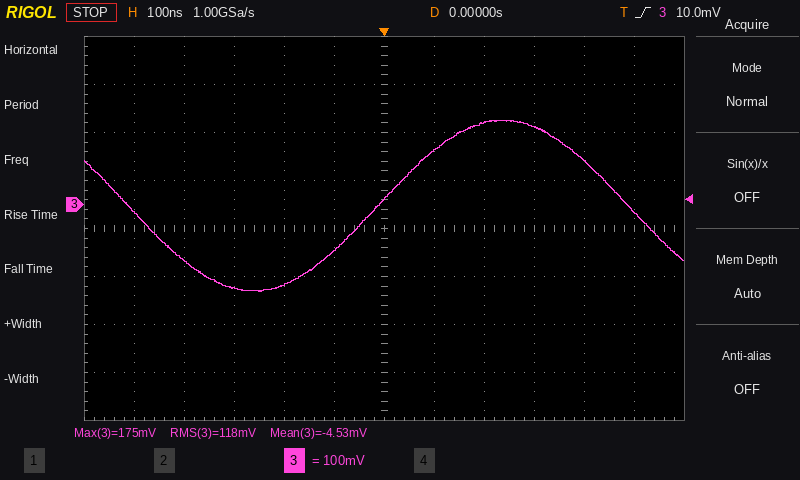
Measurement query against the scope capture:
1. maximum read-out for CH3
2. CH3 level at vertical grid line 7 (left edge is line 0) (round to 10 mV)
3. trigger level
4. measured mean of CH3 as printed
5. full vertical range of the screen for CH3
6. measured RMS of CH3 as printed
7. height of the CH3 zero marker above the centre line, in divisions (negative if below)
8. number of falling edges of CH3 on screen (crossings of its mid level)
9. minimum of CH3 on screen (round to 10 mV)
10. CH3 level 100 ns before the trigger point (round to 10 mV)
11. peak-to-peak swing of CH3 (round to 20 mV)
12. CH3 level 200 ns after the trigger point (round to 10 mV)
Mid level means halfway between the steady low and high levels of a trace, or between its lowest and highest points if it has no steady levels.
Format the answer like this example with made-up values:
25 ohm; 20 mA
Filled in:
175 mV; 110 mV; 10.0 mV; -4.53 mV; 800 mV; 118 mV; +0.5 div; 2; -180 mV; -100 mV; 360 mV; 170 mV
